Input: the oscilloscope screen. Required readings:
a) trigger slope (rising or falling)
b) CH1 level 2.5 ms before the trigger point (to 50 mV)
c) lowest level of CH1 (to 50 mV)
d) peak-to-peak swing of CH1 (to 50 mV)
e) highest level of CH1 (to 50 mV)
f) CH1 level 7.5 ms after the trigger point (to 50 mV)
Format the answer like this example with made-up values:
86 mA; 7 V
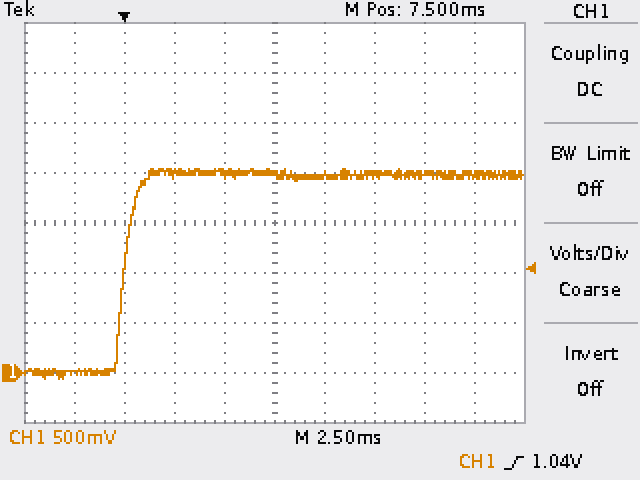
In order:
rising; 0 mV; -50 mV; 2.10 V; 2.05 V; 2.00 V
